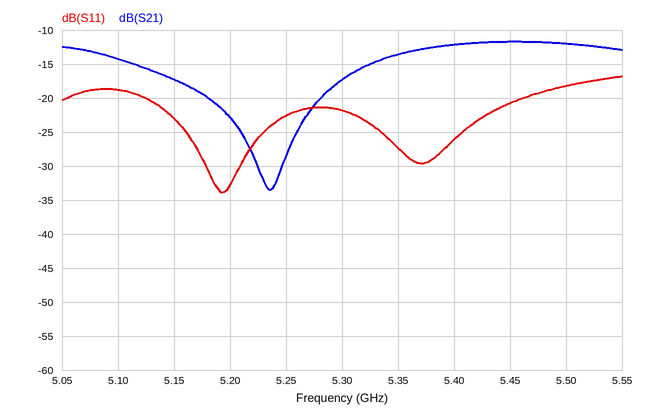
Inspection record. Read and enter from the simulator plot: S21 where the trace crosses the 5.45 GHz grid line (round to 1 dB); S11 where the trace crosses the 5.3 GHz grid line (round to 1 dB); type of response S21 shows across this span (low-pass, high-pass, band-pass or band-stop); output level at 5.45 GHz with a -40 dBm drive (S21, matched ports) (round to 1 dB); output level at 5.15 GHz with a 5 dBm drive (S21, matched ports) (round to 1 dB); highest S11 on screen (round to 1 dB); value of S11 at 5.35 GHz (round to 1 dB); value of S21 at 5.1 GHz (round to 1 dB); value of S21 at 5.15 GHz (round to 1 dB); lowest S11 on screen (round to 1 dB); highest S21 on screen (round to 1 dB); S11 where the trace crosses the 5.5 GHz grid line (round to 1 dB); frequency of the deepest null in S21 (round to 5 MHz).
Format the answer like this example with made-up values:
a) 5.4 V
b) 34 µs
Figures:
a) -12 dB
b) -22 dB
c) band-stop
d) -52 dBm
e) -12 dBm
f) -17 dB
g) -27 dB
h) -14 dB
i) -17 dB
j) -34 dB
k) -12 dB
l) -18 dB
m) 5.235 GHz
